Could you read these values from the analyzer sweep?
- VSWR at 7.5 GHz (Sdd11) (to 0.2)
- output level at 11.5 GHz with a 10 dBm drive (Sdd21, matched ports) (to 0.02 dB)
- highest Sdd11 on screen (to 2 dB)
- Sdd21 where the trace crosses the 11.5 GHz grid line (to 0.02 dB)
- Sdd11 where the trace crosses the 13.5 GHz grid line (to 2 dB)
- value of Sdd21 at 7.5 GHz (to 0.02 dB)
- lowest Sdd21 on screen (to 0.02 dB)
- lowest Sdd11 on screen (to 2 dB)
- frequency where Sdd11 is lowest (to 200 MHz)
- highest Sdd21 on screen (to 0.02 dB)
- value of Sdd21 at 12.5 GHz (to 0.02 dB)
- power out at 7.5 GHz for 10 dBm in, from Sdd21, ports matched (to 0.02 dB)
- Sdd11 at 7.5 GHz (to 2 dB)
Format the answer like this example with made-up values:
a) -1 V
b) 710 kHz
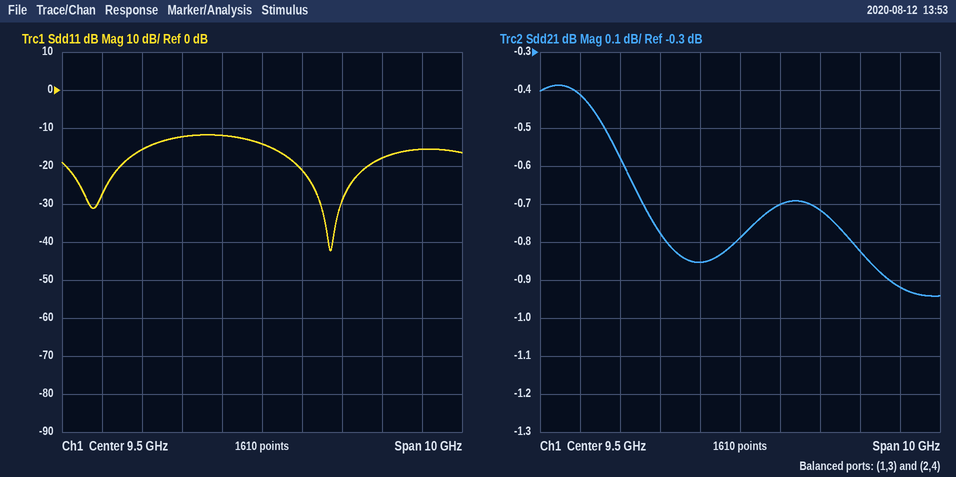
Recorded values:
a) 1.6
b) 9.28 dBm
c) -12 dB
d) -0.72 dB
e) -16 dB
f) -0.78 dB
g) -0.94 dB
h) -42 dB
i) 11.2 GHz
j) -0.38 dB
k) -0.82 dB
l) 9.22 dBm
m) -12 dB
